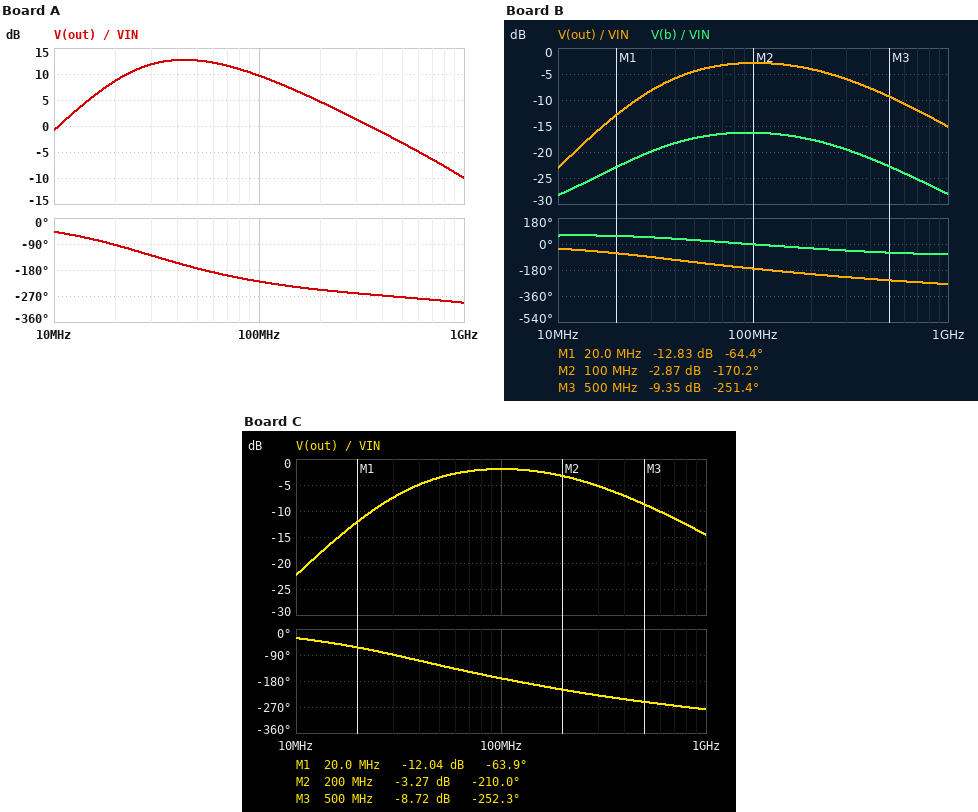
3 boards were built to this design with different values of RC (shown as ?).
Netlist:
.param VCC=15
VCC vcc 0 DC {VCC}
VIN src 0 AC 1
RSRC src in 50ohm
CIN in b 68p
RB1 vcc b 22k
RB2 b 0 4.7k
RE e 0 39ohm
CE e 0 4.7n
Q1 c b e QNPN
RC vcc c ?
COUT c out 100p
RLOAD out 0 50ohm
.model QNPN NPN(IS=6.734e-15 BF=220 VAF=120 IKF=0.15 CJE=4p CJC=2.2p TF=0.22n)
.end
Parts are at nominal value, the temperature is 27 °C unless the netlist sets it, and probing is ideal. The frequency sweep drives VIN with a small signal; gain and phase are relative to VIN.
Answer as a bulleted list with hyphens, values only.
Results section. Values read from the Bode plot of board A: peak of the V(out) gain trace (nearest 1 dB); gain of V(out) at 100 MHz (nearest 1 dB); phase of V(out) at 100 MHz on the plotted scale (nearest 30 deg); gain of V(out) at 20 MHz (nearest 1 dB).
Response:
- 13 dB
- 10 dB
- -210 deg
- 9 dB
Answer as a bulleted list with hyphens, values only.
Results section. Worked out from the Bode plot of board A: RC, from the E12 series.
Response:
- 470 Ω
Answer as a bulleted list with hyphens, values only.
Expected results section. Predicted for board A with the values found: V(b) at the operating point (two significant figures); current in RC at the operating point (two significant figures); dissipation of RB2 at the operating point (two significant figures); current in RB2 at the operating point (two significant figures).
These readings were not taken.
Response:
- 1.9 V
- 29 mA
- 770 µW
- 400 µA
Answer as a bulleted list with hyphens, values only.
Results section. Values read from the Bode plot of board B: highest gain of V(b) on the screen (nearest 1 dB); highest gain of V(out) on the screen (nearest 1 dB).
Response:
- -16 dB
- -3 dB
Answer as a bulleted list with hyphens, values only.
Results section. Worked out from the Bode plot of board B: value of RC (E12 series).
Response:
- 2.2 kΩ
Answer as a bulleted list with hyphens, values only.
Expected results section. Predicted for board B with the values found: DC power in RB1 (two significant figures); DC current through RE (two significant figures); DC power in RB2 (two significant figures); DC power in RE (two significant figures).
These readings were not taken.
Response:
- 8.9 mW
- 7.1 mA
- 210 µW
- 2.0 mW
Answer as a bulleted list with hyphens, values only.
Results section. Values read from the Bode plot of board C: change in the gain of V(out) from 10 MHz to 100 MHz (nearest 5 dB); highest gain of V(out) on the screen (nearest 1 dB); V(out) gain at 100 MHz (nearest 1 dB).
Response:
- 20 dB
- -2 dB
- -2 dB
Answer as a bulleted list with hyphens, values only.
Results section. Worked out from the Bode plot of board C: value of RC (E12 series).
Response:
- 1.8 kΩ
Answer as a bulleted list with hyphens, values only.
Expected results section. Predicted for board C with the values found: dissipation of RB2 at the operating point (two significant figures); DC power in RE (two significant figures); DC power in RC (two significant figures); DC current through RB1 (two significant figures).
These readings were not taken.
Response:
- 240 µW
- 2.8 mW
- 120 mW
- 630 µA
